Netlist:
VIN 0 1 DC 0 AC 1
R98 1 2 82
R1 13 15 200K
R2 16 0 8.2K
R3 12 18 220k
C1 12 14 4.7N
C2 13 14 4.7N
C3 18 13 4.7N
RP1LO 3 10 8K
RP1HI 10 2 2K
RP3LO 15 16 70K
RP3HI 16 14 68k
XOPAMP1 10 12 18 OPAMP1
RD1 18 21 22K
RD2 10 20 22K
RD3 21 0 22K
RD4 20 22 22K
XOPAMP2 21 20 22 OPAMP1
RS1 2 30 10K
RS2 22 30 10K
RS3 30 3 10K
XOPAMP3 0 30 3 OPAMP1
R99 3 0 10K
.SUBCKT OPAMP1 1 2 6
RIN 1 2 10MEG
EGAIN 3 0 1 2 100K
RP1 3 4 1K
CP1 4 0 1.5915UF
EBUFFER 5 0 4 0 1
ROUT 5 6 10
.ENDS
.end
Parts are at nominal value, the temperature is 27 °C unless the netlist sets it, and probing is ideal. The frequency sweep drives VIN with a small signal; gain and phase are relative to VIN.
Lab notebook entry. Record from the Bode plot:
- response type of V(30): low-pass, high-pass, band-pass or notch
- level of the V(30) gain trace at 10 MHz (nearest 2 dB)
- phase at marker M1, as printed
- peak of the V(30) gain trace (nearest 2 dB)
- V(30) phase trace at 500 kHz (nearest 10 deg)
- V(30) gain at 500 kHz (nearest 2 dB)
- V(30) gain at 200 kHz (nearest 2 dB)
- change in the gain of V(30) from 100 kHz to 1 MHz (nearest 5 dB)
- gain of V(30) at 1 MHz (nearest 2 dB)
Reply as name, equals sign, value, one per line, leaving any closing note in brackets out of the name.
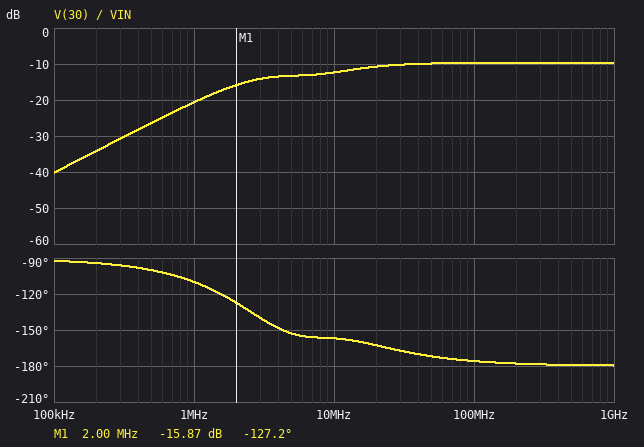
response type of V(30): low-pass, high-pass, band-pass or notch = high-pass
level of the V(30) gain trace at 10 MHz = -12 dB
phase at marker M1, as printed = -127.2 deg
peak of the V(30) gain trace = -10 dB
V(30) phase trace at 500 kHz = -100 deg
V(30) gain at 500 kHz = -26 dB
V(30) gain at 200 kHz = -34 dB
change in the gain of V(30) from 100 kHz to 1 MHz = 20 dB
gain of V(30) at 1 MHz = -20 dB
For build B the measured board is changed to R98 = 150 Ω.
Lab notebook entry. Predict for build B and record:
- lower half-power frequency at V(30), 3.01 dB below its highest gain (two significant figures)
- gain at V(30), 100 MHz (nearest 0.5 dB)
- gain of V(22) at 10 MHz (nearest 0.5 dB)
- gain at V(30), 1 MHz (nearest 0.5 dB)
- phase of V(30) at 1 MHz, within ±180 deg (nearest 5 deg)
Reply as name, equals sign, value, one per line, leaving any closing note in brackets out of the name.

lower half-power frequency at V(30), 3.01 dB below its highest gain = 8.7 MHz
gain at V(30), 100 MHz = -10.0 dB
gain of V(22) at 10 MHz = -13.0 dB
gain at V(30), 1 MHz = -21.0 dB
phase of V(30) at 1 MHz, within ±180 deg = -110 deg
